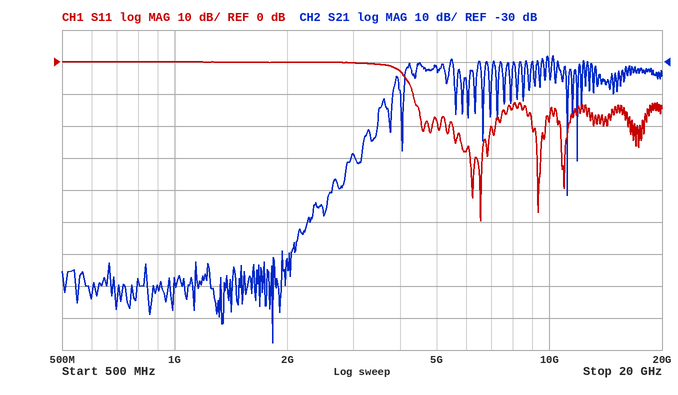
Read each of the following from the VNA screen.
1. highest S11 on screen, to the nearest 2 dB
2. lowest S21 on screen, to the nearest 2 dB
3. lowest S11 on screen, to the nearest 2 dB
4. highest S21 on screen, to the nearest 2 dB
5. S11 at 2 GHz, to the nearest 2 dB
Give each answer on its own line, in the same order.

0 dB
-118 dB
-50 dB
-28 dB
0 dB
